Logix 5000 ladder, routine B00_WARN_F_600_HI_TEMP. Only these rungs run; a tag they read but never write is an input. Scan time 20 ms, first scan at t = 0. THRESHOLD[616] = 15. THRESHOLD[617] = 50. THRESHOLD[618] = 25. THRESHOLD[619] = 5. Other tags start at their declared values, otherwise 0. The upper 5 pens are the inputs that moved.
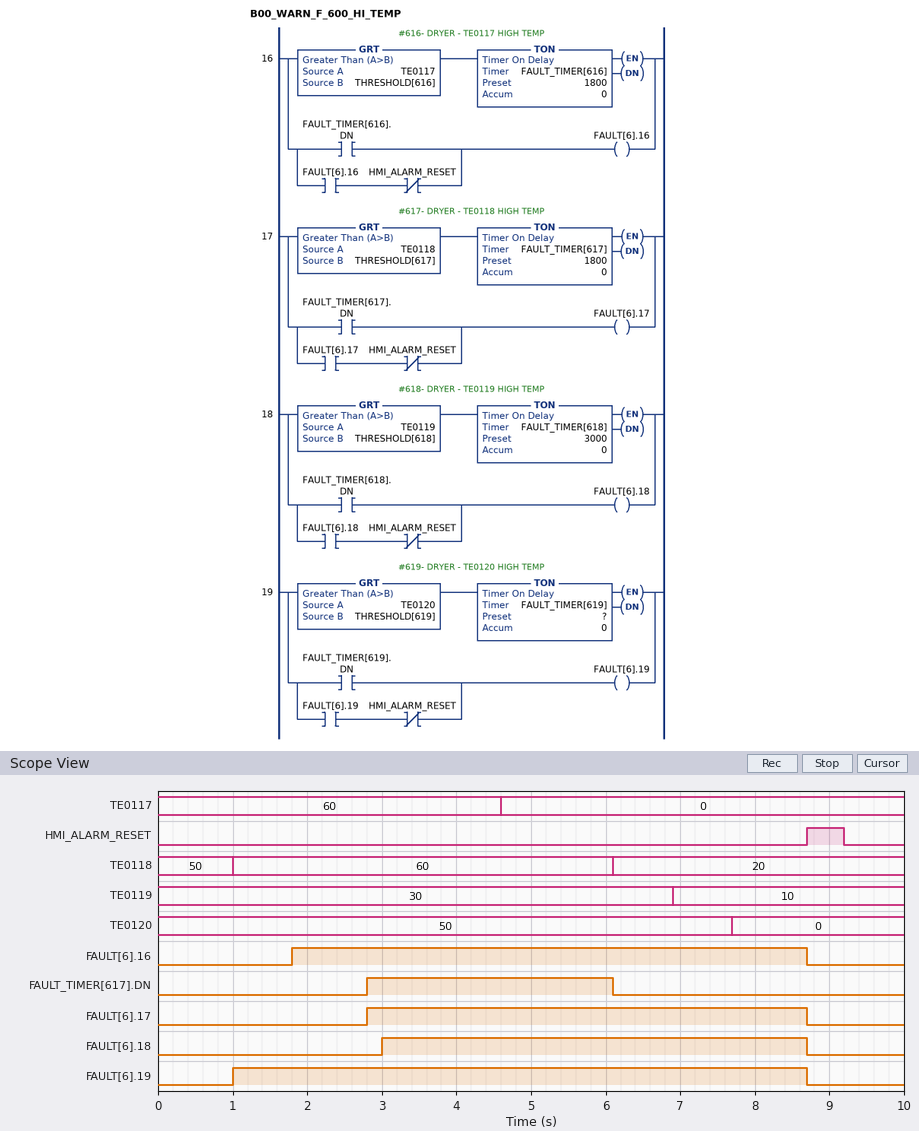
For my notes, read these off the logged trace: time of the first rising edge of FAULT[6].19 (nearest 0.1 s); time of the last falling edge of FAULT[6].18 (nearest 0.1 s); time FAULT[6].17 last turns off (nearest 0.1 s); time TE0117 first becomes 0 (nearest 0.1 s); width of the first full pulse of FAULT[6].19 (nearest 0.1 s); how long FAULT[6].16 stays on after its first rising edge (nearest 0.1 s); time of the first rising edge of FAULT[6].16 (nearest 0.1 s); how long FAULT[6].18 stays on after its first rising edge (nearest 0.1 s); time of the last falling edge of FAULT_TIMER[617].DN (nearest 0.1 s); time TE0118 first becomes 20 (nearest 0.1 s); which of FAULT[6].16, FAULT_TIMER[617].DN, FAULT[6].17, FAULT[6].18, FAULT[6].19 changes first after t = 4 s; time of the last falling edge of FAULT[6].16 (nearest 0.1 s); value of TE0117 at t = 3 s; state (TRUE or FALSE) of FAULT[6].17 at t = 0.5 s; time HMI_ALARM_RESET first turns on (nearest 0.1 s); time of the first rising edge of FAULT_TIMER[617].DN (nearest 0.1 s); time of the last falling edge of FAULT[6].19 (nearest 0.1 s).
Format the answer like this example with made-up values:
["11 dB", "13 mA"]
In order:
["1.0 s", "8.7 s", "8.7 s", "4.6 s", "7.7 s", "6.9 s", "1.8 s", "5.7 s", "6.1 s", "6.1 s", "FAULT_TIMER[617].DN", "8.7 s", "60", "FALSE", "8.7 s", "2.8 s", "8.7 s"]
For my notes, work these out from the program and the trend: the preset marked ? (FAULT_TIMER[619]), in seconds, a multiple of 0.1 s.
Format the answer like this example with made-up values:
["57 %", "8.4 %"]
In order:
["1.0 s"]
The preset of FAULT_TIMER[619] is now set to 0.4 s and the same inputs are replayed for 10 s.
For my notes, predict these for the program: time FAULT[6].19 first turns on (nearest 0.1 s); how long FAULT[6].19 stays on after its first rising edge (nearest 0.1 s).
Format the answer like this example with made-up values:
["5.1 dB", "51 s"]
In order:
["0.4 s", "8.3 s"]
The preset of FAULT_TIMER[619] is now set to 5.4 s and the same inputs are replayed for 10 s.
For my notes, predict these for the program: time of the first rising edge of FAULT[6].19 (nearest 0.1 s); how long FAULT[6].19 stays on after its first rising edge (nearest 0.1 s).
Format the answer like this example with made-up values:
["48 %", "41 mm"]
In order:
["5.4 s", "3.3 s"]
